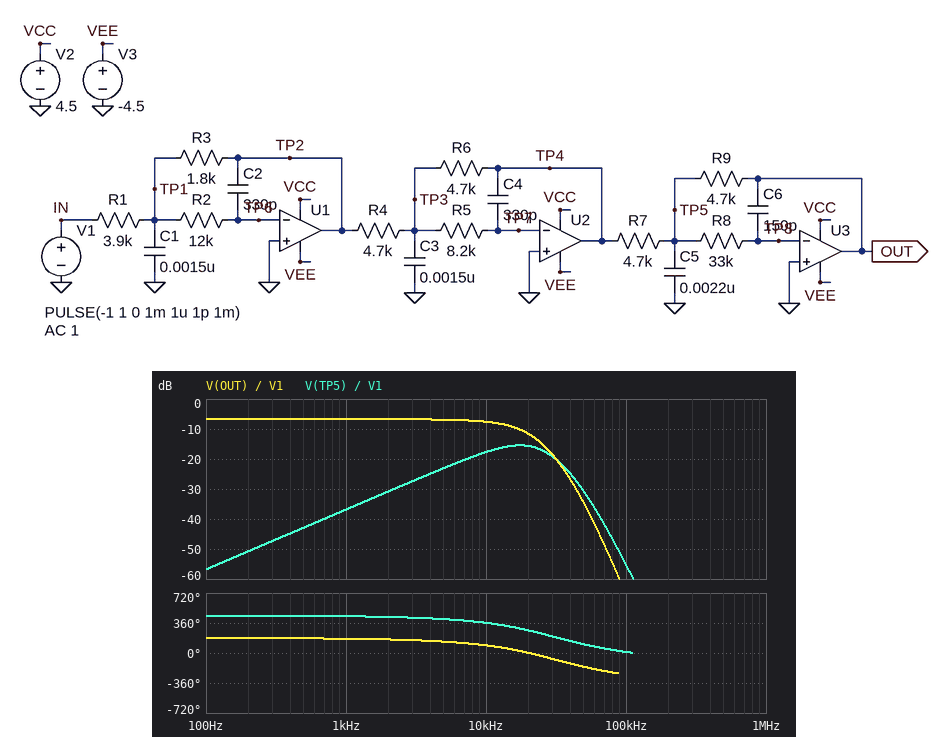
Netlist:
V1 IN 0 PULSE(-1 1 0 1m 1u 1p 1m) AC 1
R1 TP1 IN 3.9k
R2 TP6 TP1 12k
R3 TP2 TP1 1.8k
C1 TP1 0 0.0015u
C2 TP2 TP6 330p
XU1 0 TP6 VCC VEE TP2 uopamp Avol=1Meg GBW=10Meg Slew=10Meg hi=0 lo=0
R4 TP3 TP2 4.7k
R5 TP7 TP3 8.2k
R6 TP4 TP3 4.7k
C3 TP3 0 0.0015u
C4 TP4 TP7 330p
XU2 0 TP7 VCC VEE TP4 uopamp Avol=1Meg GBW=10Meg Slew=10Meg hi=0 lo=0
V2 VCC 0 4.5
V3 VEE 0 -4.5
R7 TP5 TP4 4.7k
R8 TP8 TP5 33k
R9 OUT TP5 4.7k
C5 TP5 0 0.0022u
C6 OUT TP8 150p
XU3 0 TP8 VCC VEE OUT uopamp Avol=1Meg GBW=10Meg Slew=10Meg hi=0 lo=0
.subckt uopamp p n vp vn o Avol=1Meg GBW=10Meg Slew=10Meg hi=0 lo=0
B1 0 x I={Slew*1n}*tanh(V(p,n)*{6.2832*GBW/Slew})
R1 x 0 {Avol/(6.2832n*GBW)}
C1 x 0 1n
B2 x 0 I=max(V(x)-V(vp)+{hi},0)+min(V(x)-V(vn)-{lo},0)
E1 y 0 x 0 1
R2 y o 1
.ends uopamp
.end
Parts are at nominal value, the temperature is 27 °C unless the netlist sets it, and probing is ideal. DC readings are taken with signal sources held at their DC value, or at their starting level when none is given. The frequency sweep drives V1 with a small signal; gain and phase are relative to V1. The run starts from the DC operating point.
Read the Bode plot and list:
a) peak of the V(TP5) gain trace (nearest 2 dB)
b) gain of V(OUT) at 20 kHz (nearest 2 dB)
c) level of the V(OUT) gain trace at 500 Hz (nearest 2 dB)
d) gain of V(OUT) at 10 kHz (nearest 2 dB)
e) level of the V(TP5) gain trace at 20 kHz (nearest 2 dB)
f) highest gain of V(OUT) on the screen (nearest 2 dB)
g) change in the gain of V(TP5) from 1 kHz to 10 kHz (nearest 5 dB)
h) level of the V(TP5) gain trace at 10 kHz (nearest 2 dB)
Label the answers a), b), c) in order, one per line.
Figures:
a) -16 dB
b) -12 dB
c) -6 dB
d) -8 dB
e) -16 dB
f) -6 dB
g) 20 dB
h) -18 dB
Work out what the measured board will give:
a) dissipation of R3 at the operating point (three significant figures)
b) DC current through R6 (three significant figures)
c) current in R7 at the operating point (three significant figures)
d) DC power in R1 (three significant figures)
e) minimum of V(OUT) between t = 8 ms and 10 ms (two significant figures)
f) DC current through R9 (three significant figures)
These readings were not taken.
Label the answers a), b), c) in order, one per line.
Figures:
a) 118 µW
b) 98.2 µA
c) 98.2 µA
d) 256 µW
e) -440 mV
f) 98.2 µA
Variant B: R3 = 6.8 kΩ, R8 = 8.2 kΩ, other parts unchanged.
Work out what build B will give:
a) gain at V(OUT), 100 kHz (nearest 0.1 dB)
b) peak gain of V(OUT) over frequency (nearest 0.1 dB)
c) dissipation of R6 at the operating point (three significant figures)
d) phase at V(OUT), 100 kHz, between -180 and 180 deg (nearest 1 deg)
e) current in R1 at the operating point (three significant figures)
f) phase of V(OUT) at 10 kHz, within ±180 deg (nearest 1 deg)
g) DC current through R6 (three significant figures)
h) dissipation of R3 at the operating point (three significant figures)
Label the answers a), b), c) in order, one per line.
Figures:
a) -51.0 dB
b) 4.8 dB
c) 647 µW
d) 87 deg
e) 256 µA
f) 98 deg
g) 371 µA
h) 447 µW
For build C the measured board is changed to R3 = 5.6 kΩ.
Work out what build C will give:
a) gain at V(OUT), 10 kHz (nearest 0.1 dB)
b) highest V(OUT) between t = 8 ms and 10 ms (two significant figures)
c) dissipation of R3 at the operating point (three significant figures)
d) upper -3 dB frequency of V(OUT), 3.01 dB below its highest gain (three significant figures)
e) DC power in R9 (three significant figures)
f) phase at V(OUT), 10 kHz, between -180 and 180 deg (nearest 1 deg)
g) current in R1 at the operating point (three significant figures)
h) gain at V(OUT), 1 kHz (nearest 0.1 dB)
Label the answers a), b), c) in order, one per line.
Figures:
a) 1.5 dB
b) 1.4 V
c) 368 µW
d) 13.4 kHz
e) 439 µW
f) 75 deg
g) 256 µA
h) 3.1 dB
